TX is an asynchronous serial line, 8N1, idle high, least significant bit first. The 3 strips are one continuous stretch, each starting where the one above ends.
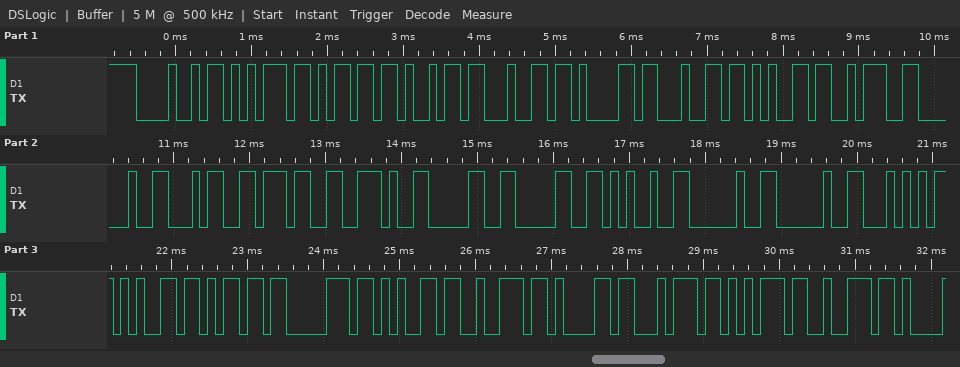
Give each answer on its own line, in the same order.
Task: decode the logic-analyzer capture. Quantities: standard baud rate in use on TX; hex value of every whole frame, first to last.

9600 baud
0x48 0x75 0x6D 0x69 0x64 0x61 0x64 0x65 0x3A 0x20 0x34 0x37 0x2E 0x30 0x30 0x25 0x20 0x20 0x54 0x65 0x6D 0x70 0x65 0x72 0x61 0x74 0x75 0x72
